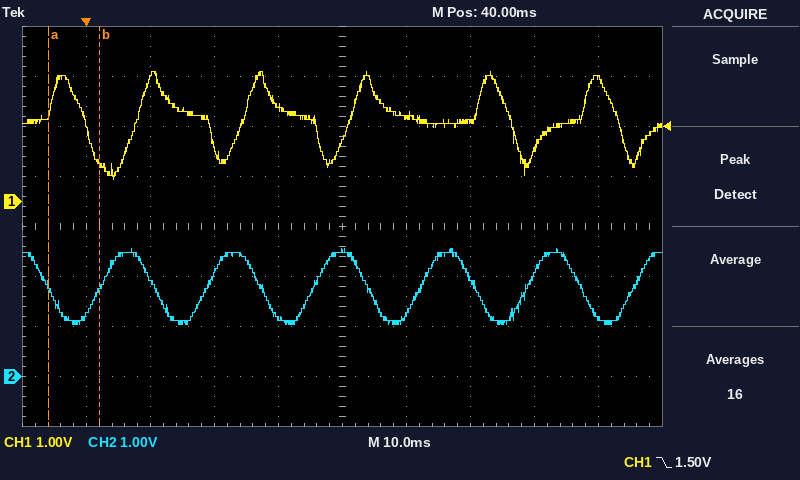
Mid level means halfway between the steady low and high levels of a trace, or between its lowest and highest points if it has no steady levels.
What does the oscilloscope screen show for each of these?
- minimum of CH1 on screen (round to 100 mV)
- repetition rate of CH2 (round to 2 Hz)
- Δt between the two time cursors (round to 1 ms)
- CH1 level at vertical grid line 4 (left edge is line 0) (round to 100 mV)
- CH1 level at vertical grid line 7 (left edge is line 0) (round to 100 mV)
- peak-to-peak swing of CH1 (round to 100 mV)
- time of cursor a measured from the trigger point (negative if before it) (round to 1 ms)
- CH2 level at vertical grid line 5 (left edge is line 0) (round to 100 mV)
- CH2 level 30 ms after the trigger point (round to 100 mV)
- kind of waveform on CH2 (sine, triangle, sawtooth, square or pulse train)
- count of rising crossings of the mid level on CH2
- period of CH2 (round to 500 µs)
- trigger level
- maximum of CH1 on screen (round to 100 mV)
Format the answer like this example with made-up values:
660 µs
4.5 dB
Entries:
400 mV
60 Hz
8 ms
1.9 V
1.6 V
2.2 V
-6 ms
2.5 V
1.2 V
sine
6
16.5 ms
1.50 V
2.6 V
